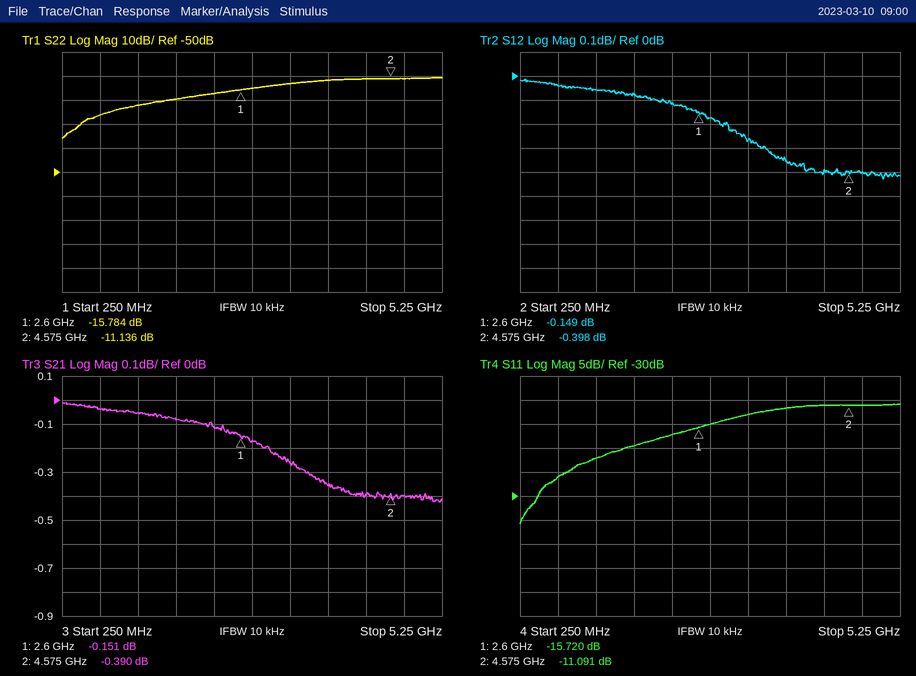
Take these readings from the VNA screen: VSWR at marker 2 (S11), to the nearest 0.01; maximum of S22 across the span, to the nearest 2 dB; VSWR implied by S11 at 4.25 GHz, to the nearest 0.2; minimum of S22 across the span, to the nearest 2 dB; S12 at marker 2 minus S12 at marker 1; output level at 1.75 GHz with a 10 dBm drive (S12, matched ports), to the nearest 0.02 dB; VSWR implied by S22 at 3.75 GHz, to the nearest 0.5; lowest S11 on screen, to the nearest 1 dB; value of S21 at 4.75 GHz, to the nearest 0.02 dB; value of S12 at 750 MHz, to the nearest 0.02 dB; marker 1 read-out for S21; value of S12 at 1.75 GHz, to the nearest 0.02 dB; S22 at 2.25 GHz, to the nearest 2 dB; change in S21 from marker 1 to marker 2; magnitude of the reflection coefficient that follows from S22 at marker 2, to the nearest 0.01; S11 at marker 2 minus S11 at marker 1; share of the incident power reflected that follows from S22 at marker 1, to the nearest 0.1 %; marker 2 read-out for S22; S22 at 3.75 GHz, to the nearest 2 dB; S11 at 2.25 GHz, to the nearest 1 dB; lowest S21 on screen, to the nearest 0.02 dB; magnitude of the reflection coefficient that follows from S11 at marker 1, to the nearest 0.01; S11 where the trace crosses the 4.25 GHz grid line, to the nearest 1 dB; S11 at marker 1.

1.77
-10 dB
1.8
-36 dB
-0.249 dB
9.92 dBm
1.5
-36 dB
-0.40 dB
-0.04 dB
-0.151 dB
-0.08 dB
-18 dB
-0.239 dB
0.28
4.629 dB
2.6 %
-11.136 dB
-12 dB
-17 dB
-0.42 dB
0.16
-11 dB
-15.720 dB
